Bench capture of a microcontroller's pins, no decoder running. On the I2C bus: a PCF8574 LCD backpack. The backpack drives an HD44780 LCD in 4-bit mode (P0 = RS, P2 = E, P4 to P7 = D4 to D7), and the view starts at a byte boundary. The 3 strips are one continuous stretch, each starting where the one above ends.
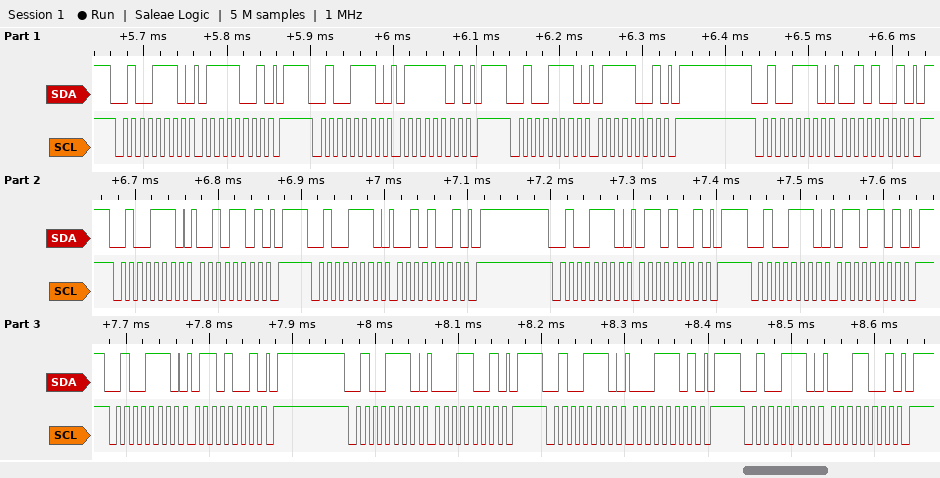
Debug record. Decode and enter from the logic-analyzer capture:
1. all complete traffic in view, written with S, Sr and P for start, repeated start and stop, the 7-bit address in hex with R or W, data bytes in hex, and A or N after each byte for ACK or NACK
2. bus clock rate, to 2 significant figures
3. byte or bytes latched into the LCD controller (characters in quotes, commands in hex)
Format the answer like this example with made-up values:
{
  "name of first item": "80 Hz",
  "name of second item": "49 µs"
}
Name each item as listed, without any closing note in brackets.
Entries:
{
  "all complete traffic in view, written with S, Sr and P for start, repeated start and stop, the 7-bit address in hex with R or W, data bytes in hex, and A or N after each byte for ACK or NACK": "S 27W A 79 A P S 27W A 7D A P S 27W A 79 A P S 27W A 29 A P S 27W A 2D A P S 27W A 29 A P S 27W A 69 A P S 27W A 6D A P S 27W A 69 A P S 27W A 19 A P S 27W A 1D A P S 27W A 19 A P",
  "bus clock rate, to 2 significant figures": "100 kHz",
  "byte or bytes latched into the LCD controller": "'r' 'a'"
}
